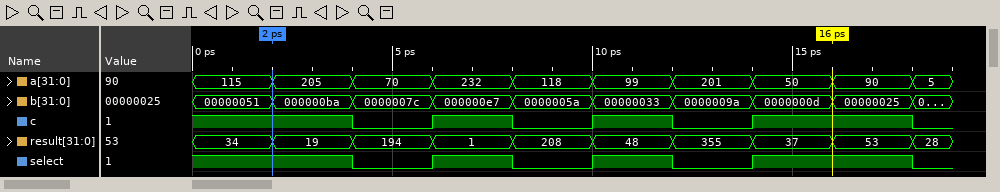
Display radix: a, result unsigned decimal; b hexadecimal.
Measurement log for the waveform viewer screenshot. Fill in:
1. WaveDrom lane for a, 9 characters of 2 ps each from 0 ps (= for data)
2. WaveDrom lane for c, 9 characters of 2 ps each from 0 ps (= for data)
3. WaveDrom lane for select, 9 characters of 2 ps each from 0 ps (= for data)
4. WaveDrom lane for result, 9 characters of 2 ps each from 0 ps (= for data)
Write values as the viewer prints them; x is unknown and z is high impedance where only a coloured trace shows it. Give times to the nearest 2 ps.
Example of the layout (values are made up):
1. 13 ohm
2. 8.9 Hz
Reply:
1. {name: 'a', wave: '=========', data: '115 205 70 232 118 99 201 50 90'}
2. {name: 'c', wave: '1.010101.'}
3. {name: 'select', wave: '1.010101.'}
4. {name: 'result', wave: '=========', data: '34 19 194 1 208 48 355 37 53'}
